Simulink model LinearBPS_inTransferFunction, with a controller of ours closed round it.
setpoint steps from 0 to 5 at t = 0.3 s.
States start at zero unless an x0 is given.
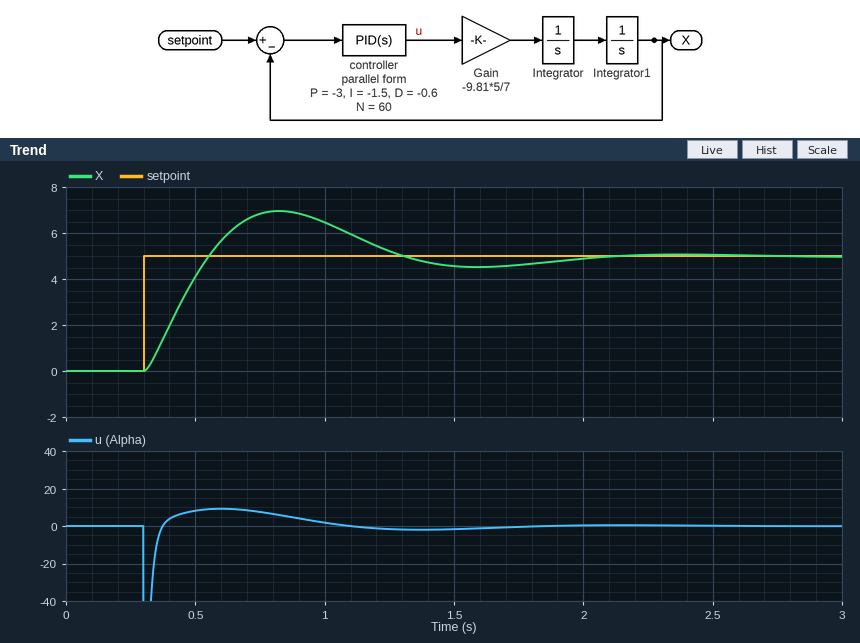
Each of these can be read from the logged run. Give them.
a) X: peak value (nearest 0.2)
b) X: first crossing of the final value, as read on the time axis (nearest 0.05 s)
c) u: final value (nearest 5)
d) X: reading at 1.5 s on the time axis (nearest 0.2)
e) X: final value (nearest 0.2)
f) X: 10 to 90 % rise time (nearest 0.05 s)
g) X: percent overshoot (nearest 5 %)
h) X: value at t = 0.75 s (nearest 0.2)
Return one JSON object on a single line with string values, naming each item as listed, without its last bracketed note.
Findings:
{"X: peak value": "7.0", "X: first crossing of the final value, as read on the time axis": "0.55 s", "u: final value": "0", "X: reading at 1.5 s on the time axis": "4.6", "X: final value": "5.0", "X: 10 to 90 % rise time": "0.20 s", "X: percent overshoot": "40 %", "X: value at t = 0.75 s": "6.8"}
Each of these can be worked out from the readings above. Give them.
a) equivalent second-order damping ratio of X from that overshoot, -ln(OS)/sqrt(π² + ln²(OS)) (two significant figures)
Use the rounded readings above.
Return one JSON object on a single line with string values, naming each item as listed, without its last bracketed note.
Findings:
{"equivalent second-order damping ratio of X from that overshoot, -ln(OS)/sqrt(π² + ln²(OS))": "0.28"}
